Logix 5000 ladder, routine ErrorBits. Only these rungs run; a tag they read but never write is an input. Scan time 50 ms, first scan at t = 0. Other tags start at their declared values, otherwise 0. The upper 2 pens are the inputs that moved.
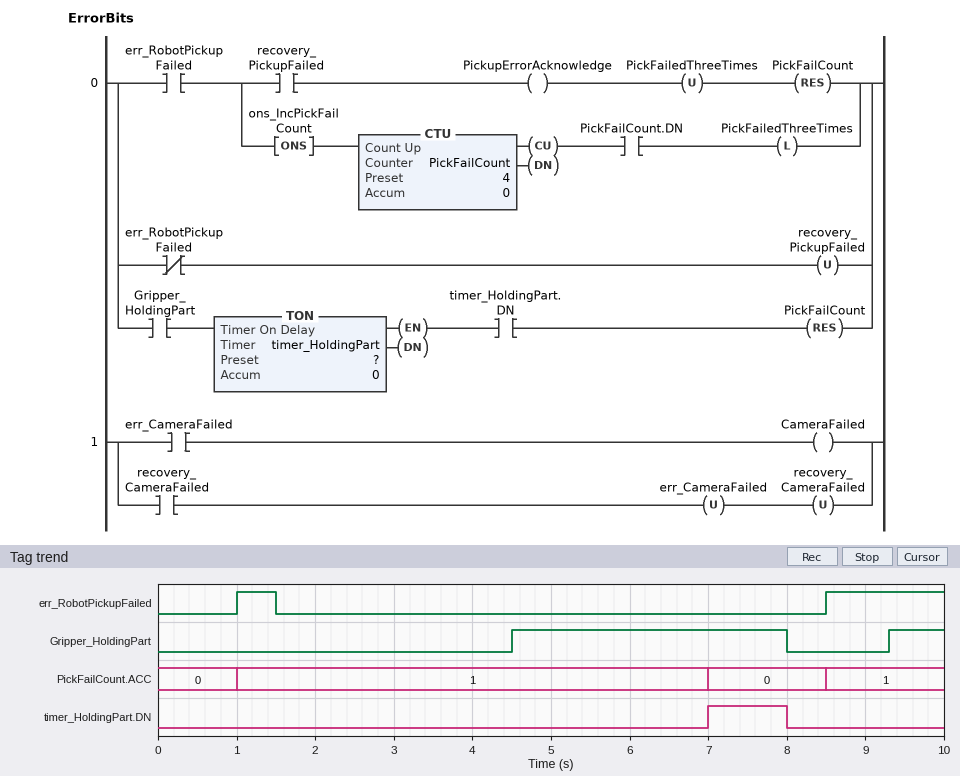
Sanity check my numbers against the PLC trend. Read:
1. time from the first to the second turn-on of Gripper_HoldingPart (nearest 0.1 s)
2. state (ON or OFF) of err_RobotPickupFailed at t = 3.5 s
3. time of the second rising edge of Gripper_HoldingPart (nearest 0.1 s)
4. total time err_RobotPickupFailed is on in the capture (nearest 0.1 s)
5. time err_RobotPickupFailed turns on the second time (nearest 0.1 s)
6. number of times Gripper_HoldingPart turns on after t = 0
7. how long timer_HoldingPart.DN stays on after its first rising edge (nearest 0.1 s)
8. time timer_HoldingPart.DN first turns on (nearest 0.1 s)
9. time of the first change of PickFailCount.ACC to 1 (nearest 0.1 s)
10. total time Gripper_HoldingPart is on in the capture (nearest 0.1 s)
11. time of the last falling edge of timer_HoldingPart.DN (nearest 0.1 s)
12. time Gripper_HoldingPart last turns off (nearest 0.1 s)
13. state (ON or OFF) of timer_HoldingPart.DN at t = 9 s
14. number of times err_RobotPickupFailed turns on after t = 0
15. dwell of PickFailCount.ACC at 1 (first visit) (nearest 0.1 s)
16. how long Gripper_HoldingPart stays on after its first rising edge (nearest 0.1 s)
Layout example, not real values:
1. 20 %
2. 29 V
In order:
1. 4.8 s
2. OFF
3. 9.3 s
4. 2.0 s
5. 8.5 s
6. 2
7. 1.0 s
8. 7.0 s
9. 1.0 s
10. 4.2 s
11. 8.0 s
12. 8.0 s
13. OFF
14. 2
15. 6.0 s
16. 3.5 s
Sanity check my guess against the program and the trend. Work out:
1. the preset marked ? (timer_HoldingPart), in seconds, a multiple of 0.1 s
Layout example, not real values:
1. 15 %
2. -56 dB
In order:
1. 2.5 s
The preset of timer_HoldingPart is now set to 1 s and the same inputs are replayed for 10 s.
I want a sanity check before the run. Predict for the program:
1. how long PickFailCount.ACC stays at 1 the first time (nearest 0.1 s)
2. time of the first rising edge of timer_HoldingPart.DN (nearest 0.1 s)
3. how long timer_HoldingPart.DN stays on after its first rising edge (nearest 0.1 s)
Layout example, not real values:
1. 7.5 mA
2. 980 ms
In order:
1. 4.5 s
2. 5.5 s
3. 2.5 s
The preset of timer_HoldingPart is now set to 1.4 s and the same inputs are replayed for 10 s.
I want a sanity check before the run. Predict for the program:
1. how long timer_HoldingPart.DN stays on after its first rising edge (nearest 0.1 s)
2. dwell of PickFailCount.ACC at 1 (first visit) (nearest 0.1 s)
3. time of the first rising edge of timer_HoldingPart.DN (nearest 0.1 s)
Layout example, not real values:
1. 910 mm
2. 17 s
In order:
1. 2.1 s
2. 4.9 s
3. 5.9 s
